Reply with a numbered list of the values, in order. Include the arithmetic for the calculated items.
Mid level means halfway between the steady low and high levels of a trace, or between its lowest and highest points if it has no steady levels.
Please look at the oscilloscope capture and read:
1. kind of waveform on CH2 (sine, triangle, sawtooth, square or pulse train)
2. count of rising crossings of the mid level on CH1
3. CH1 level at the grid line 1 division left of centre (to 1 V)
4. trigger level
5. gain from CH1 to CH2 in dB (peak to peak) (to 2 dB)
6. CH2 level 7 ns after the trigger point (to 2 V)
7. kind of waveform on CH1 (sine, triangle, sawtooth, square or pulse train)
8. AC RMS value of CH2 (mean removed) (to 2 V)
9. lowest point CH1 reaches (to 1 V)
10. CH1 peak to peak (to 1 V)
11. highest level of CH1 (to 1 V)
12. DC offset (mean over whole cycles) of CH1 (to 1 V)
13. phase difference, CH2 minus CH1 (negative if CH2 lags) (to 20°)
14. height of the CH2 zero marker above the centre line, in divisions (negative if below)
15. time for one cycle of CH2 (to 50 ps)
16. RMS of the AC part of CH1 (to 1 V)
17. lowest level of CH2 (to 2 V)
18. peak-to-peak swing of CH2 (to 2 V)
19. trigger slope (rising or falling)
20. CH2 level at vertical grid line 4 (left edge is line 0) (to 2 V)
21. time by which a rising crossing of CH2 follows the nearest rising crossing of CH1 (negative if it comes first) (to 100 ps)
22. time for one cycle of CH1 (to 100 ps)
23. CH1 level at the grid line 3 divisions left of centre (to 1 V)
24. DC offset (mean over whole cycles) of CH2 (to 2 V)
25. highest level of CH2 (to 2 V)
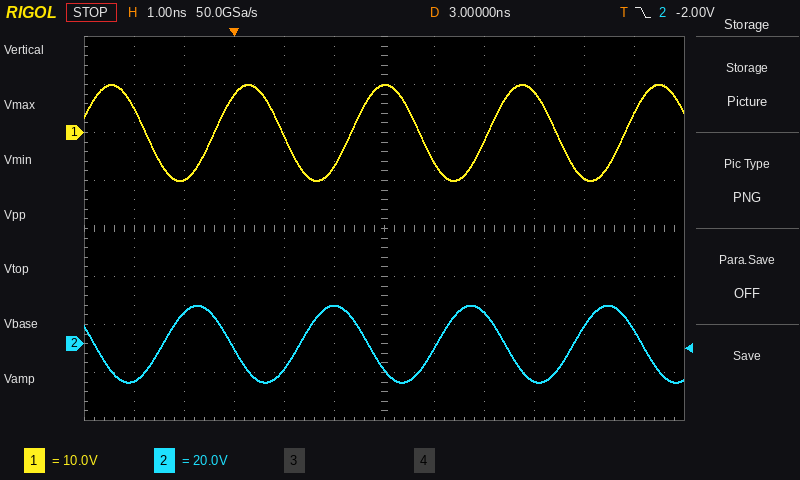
1. sine
2. 4
3. -7 V
4. -2.00 V
5. 20 log10(32 V / 20 V) ≈ 4 dB
6. 8 V
7. sine
8. 32 V / (2√2) ≈ 11.3 V, so 12 V to the nearest 2 V
9. -10 V
10. 10 V − (-10 V) = 20 V
11. 10 V
12. (10 V + (-10 V)) / 2 ≈ 0 V
13. −360° × (-1.0 ns) / 2.7 ns ≈ +133°, so +140° to the nearest 20°
14. -2.4 div
15. 2.75 ns
16. 20 V / (2√2) ≈ 7 V
17. -16 V
18. 16 V − (-16 V) = 32 V
19. falling
20. -10 V
21. -1.0 ns
22. 2.7 ns
23. 8 V
24. (16 V + (-16 V)) / 2 ≈ 0 V
25. 16 V
